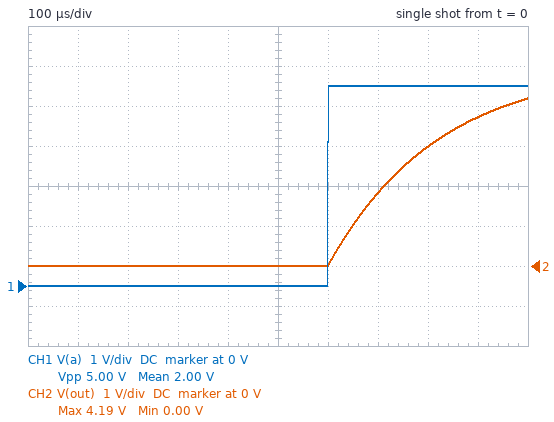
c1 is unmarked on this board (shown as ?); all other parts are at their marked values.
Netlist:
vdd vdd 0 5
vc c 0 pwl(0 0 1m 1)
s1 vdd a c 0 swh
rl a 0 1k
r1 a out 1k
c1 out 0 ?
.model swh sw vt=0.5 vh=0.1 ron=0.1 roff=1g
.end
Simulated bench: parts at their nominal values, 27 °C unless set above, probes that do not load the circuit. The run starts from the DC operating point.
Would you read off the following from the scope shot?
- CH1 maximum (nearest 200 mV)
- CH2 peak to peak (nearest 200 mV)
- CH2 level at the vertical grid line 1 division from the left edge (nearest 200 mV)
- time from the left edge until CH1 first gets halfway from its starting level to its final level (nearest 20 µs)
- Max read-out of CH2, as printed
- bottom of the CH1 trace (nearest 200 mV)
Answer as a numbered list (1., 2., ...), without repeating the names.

1. 5.0 V
2. 4.2 V
3. 0 V
4. 600 µs
5. 4.19 V
6. 0 V
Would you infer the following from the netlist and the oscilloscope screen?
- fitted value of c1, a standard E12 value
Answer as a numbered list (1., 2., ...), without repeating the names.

1. 220 nF
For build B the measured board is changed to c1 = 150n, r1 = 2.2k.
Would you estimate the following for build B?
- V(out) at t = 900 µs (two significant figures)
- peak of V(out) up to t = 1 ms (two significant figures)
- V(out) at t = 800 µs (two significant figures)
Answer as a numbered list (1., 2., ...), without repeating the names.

1. 3.0 V
2. 3.5 V
3. 2.3 V
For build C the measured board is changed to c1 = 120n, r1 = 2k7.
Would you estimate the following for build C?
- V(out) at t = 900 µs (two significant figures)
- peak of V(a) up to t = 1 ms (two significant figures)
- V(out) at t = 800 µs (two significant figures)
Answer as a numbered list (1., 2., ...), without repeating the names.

1. 3.0 V
2. 5.0 V
3. 2.3 V
